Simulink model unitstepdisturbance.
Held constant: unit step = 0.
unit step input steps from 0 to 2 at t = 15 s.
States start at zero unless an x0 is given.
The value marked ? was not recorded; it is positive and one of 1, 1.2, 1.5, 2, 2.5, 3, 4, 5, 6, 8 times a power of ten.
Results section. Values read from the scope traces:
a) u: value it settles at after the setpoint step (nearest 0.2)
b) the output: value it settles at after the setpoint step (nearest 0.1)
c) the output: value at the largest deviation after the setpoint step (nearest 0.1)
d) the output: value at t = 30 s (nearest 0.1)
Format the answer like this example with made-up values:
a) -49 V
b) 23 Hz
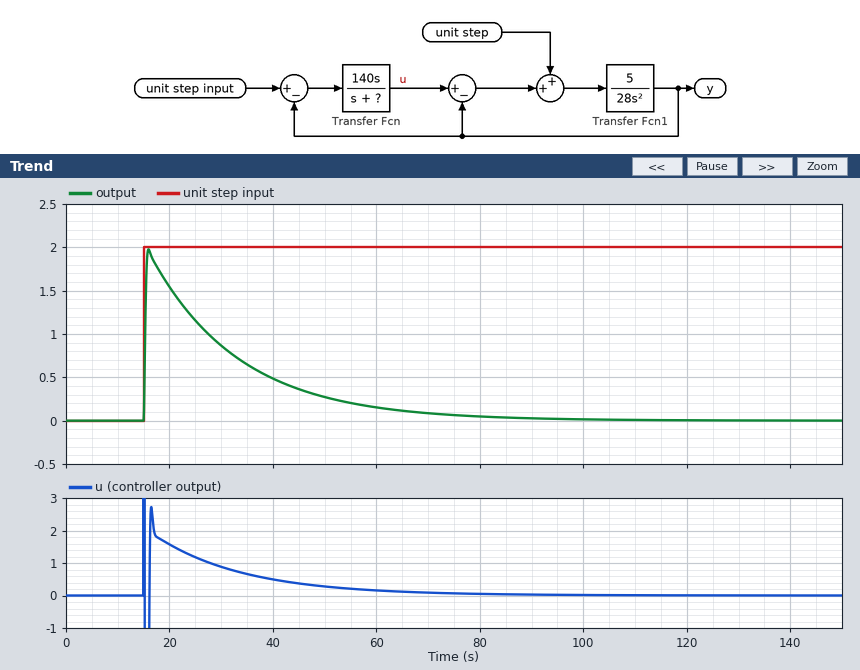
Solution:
a) 0.0
b) 0.0
c) 2.0
d) 0.9
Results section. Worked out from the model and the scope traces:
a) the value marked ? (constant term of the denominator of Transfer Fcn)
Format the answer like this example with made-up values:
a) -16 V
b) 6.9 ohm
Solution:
a) 8
